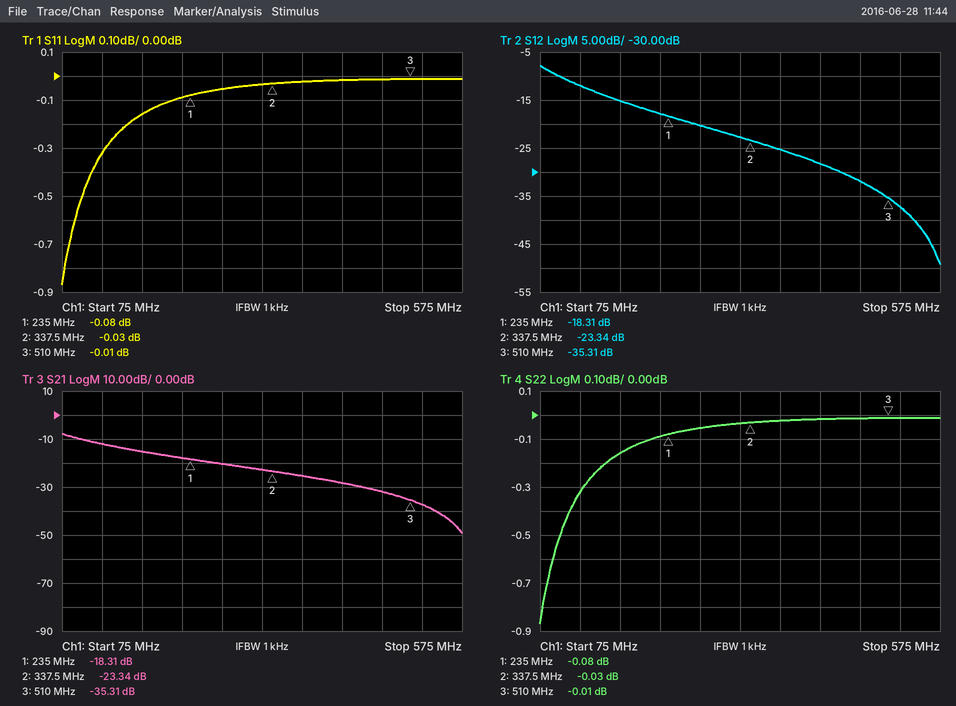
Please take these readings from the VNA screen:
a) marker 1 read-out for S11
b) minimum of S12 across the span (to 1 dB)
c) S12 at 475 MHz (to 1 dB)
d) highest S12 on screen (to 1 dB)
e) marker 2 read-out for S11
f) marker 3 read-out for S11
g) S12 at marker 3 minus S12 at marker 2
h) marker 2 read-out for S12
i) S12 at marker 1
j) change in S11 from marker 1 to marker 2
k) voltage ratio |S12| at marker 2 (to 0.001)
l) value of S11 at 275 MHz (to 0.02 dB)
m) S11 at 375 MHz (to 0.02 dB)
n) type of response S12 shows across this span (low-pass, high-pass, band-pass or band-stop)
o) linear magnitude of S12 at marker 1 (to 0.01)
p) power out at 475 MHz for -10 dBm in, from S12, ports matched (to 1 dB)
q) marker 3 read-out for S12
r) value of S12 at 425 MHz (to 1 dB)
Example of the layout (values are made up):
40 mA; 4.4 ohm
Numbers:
-0.08 dB; -49 dB; -32 dB; -8 dB; -0.03 dB; -0.01 dB; -11.97 dB; -23.34 dB; -18.31 dB; 0.05 dB; 0.068; -0.06 dB; -0.02 dB; low-pass; 0.12; -42 dBm; -35.31 dB; -28 dB
